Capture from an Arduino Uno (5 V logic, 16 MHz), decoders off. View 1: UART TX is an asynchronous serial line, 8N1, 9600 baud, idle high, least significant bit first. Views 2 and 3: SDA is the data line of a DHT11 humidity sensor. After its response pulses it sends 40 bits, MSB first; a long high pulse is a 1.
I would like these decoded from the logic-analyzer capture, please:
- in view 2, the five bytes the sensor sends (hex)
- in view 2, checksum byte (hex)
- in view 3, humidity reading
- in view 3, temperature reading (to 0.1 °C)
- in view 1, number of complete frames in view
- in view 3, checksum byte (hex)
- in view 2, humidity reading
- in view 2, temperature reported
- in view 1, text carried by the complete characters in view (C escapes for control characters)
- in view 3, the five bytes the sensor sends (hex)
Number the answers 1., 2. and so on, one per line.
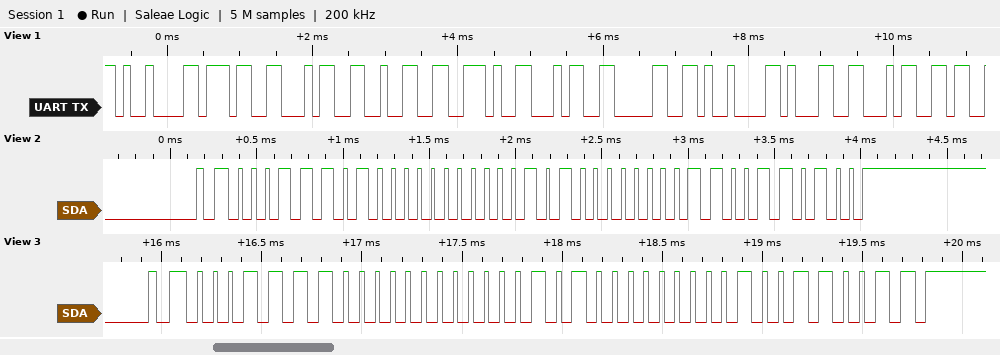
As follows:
1. 1D 00 14 03 34
2. 0x34
3. 30 %
4. 20.1 °C
5. 10
6. 0x33
7. 29 %
8. 20.3 °C
9. "\t742.40\t14"
10. 1E 00 14 01 33
